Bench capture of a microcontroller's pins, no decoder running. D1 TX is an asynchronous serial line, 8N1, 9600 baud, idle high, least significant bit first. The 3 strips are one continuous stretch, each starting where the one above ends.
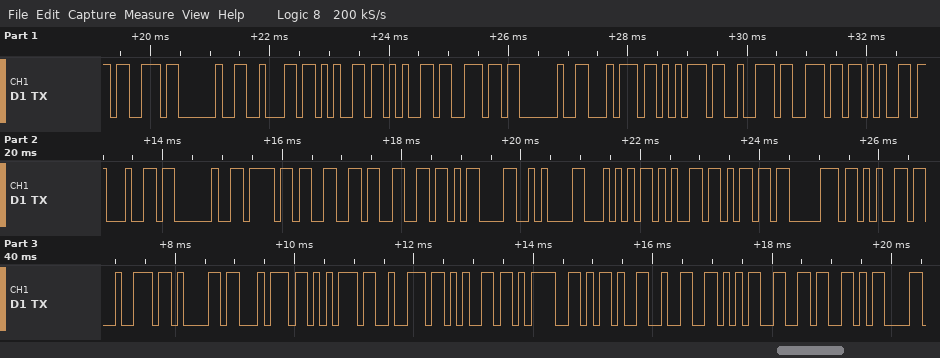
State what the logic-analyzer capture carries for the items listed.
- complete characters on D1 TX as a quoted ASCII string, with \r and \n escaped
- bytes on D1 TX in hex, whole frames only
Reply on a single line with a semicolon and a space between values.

"s been turned off\r\nTemperature=-256\r"; 73 20 62 65 65 6E 20 74 75 72 6E 65 64 20 6F 66 66 0D 0A 54 65 6D 70 65 72 61 74 75 72 65 3D 2D 32 35 36 0D
